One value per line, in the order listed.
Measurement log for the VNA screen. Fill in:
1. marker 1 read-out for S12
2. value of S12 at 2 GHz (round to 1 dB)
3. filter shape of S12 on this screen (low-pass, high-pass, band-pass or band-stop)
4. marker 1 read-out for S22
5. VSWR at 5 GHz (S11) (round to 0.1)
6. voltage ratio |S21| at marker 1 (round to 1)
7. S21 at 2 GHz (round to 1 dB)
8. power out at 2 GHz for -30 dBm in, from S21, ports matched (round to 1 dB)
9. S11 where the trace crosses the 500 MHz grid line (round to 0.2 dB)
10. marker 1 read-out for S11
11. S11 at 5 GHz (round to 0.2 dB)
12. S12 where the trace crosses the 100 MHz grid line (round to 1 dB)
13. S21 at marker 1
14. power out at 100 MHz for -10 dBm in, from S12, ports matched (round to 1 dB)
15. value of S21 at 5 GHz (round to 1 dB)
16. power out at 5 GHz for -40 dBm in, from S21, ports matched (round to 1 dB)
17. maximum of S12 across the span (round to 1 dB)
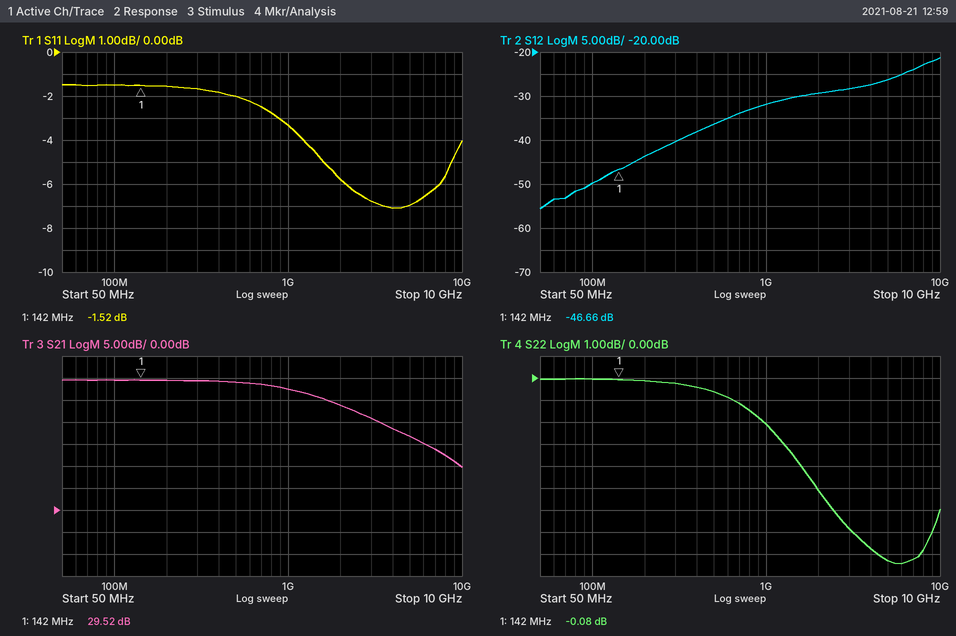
-46.66 dB
-29 dB
high-pass
-0.08 dB
2.6
30
24 dB
-6 dBm
-2.0 dB
-1.52 dB
-7.0 dB
-50 dB
29.52 dB
-60 dBm
17 dB
-23 dBm
-21 dB
